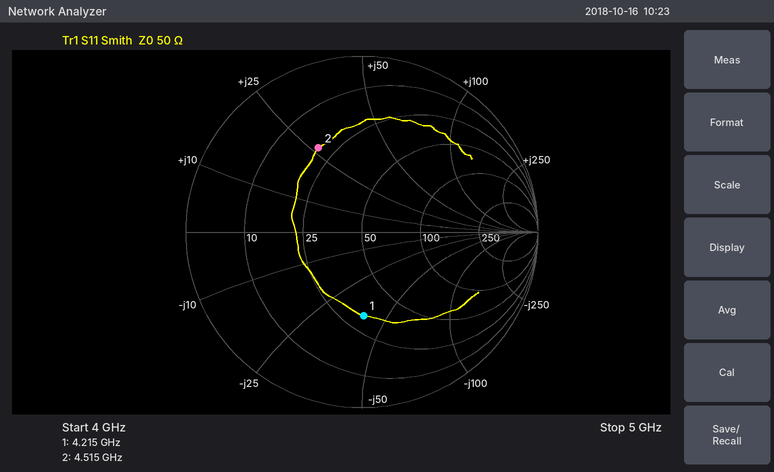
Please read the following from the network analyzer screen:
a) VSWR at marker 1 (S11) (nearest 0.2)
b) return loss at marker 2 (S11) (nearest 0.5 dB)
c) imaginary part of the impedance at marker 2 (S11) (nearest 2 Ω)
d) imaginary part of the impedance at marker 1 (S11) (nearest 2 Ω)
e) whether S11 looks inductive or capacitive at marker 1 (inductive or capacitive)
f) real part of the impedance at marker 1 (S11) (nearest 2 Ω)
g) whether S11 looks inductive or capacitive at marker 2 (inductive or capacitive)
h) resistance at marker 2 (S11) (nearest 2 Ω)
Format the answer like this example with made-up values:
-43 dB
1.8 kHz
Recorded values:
2.8
5.5 dB
+26 Ω
-40 Ω
capacitive
32 Ω
inductive
20 Ω
